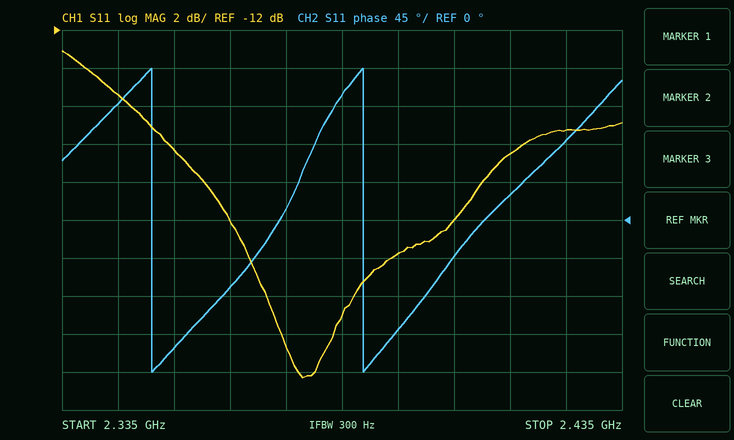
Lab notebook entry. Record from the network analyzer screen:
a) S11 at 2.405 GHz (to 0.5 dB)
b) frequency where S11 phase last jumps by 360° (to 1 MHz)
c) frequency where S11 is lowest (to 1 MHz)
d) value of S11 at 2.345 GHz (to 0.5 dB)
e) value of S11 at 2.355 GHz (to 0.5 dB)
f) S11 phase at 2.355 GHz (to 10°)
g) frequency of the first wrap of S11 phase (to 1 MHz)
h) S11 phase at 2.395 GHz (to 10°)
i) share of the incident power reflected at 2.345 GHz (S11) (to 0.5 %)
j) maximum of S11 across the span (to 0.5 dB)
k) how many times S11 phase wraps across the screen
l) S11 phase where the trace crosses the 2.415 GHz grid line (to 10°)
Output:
-22.0 dB
2.389 GHz
2.378 GHz
-15.5 dB
-18.5 dB
-150°
2.351 GHz
-130°
3.0 %
-13.0 dB
2
30°
